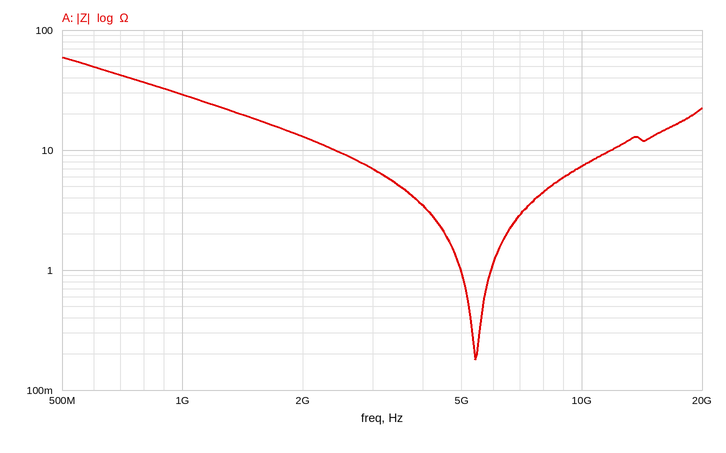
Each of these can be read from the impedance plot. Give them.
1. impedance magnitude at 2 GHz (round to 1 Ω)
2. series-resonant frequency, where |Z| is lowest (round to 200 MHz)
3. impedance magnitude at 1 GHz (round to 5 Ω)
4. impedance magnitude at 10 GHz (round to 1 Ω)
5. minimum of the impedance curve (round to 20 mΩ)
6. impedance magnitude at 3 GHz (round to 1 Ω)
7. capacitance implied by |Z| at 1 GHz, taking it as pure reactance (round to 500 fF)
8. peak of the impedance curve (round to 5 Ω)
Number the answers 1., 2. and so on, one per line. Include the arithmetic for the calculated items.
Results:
1. 13 Ω
2. 5.4 GHz
3. 30 Ω
4. 7 Ω
5. 180 mΩ
6. 7 Ω
7. C = 1/(2π × 1 GHz × 30 Ω) ≈ 5.31 pF, so 5.5 pF to the nearest 500 fF
8. 60 Ω
